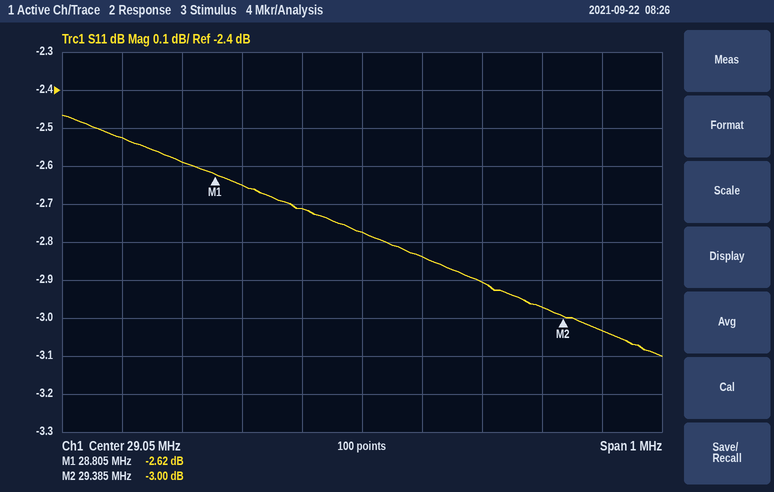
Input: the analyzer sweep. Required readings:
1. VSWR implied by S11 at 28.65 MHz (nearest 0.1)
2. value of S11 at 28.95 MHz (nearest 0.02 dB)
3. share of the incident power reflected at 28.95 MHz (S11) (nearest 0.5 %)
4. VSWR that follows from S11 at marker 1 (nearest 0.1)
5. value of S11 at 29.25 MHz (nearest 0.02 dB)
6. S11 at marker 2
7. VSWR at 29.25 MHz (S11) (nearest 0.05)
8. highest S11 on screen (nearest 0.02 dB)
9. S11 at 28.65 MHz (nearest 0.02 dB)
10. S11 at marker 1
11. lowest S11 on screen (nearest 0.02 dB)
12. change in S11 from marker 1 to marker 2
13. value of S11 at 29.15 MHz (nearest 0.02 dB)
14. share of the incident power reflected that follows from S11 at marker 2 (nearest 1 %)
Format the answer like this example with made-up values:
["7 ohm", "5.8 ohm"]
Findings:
["6.9", "-2.72 dB", "53.5 %", "6.7", "-2.90 dB", "-3.00 dB", "6.05", "-2.46 dB", "-2.52 dB", "-2.62 dB", "-3.10 dB", "-0.38 dB", "-2.84 dB", "50 %"]
